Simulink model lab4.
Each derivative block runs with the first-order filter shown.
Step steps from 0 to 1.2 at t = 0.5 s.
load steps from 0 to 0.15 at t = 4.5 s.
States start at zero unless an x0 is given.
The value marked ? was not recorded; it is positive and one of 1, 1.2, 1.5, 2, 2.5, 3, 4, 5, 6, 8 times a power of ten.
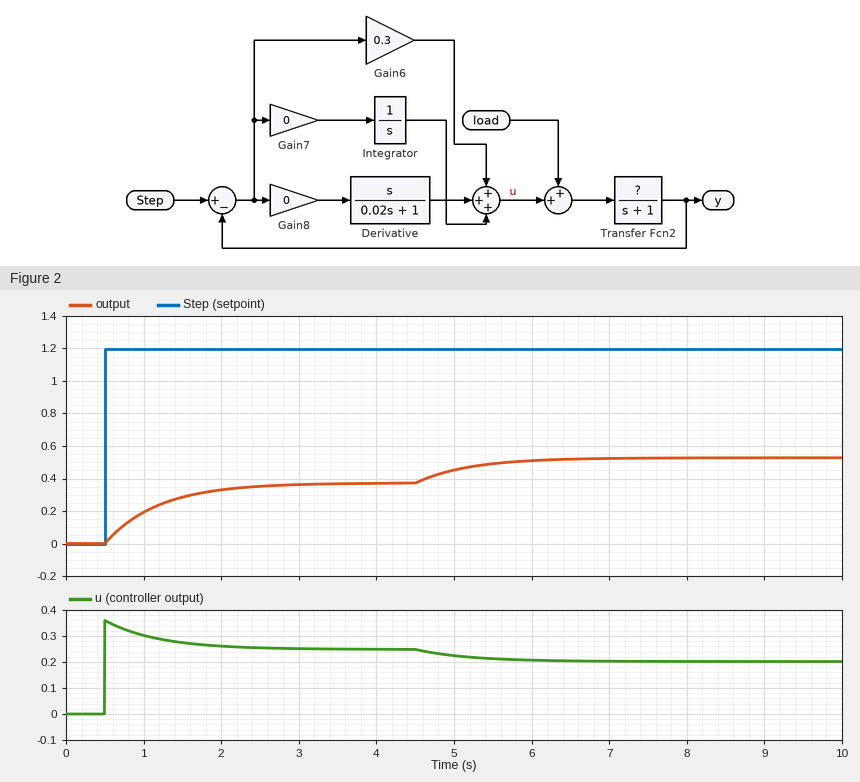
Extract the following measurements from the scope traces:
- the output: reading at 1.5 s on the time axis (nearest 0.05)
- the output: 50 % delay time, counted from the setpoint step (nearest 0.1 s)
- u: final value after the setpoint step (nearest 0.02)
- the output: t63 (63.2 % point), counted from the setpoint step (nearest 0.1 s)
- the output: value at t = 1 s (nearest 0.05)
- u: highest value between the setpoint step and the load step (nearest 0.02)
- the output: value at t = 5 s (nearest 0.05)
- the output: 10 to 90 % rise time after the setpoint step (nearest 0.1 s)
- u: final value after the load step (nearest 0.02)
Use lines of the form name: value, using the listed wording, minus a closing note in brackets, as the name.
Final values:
the output: reading at 1.5 s on the time axis: 0.30
the output: 50 % delay time, counted from the setpoint step: 0.5 s
u: final value after the setpoint step: 0.24
the output: t63 (63.2 % point), counted from the setpoint step: 0.7 s
the output: value at t = 1 s: 0.20
u: highest value between the setpoint step and the load step: 0.36
the output: value at t = 5 s: 0.45
the output: 10 to 90 % rise time after the setpoint step: 1.5 s
u: final value after the load step: 0.20
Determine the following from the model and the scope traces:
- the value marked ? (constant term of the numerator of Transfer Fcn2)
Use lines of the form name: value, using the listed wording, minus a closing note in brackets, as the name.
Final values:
the value marked ?: 1.5
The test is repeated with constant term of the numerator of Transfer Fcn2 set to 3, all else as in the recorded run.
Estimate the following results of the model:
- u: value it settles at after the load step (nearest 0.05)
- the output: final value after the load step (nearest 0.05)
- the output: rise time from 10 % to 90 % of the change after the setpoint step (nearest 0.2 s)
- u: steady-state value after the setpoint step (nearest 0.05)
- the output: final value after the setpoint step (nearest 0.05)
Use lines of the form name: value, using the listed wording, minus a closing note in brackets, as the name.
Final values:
u: value it settles at after the load step: 0.10
the output: final value after the load step: 0.80
the output: rise time from 10 % to 90 % of the change after the setpoint step: 1.2 s
u: steady-state value after the setpoint step: 0.20
the output: final value after the setpoint step: 0.55
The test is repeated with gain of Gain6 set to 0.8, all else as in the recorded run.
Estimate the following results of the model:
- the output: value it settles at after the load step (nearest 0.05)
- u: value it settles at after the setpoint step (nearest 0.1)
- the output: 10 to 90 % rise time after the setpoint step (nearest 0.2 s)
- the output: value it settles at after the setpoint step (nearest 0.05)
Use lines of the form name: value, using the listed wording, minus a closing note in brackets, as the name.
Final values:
the output: value it settles at after the load step: 0.75
u: value it settles at after the setpoint step: 0.4
the output: 10 to 90 % rise time after the setpoint step: 1.0 s
the output: value it settles at after the setpoint step: 0.65
